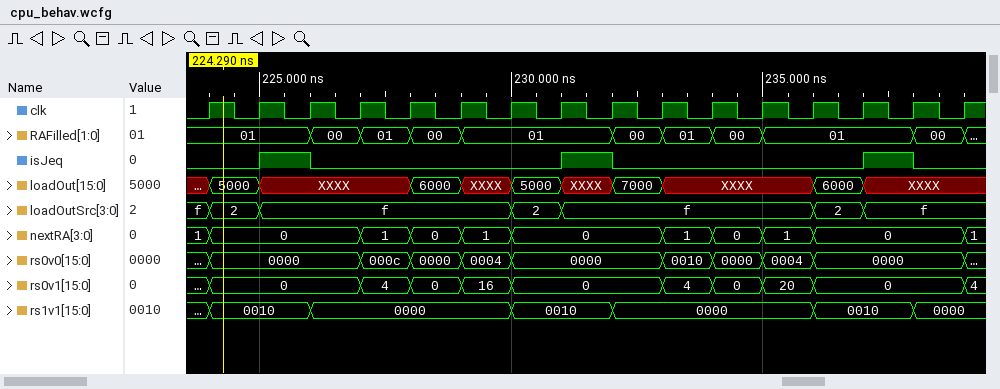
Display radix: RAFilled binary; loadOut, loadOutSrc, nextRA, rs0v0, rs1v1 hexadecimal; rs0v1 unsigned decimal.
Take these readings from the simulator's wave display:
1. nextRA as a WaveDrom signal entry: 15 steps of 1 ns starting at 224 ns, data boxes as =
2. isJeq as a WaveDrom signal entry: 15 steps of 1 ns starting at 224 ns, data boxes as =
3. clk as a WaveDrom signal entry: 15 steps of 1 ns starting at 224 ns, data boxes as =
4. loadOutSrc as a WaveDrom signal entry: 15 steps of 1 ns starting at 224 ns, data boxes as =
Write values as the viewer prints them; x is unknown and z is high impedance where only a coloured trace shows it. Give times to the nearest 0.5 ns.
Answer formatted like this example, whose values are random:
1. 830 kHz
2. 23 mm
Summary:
1. {name: 'nextRA', wave: '=..====..====..', data: '0 1 0 1 0 1 0 1 0'}
2. {name: 'isJeq', wave: '010....10....10'}
3. {name: 'clk', wave: 'p..............'}
4. {name: 'loadOutSrc', wave: '==....==....==.', data: '2 f 2 f 2 f'}
